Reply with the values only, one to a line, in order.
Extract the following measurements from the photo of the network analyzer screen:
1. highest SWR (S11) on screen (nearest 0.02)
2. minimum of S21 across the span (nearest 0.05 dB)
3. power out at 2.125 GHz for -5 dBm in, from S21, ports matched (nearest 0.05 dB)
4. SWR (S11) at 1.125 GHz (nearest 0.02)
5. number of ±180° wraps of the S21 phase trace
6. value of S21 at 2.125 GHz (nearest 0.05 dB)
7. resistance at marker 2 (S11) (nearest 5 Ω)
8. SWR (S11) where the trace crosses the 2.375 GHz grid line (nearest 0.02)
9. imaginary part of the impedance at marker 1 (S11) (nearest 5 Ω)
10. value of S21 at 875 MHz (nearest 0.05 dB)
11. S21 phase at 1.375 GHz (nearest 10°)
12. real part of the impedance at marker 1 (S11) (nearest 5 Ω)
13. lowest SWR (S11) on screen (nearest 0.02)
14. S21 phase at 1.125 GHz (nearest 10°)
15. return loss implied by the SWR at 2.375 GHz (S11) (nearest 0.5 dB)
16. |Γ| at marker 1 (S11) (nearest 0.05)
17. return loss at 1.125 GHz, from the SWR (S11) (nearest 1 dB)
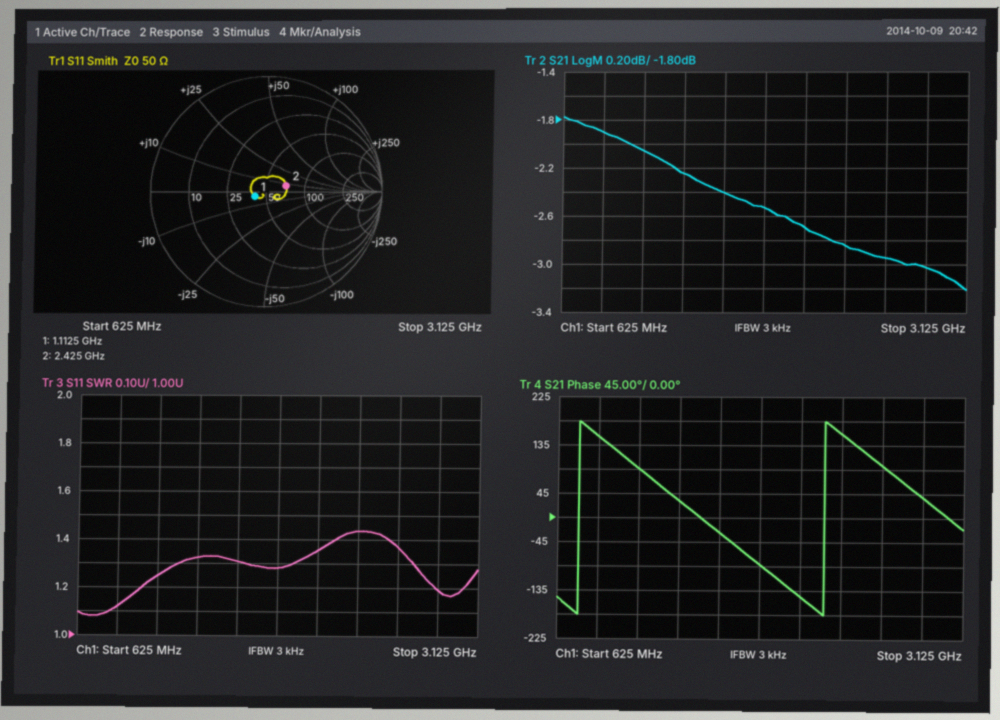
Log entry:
1.44
-3.20 dB
-7.70 dBm
1.24
2
-2.70 dB
70 Ω
1.44
-5 Ω
-1.90 dB
30°
40 Ω
1.08
90°
15.0 dB
0.10
19 dB
